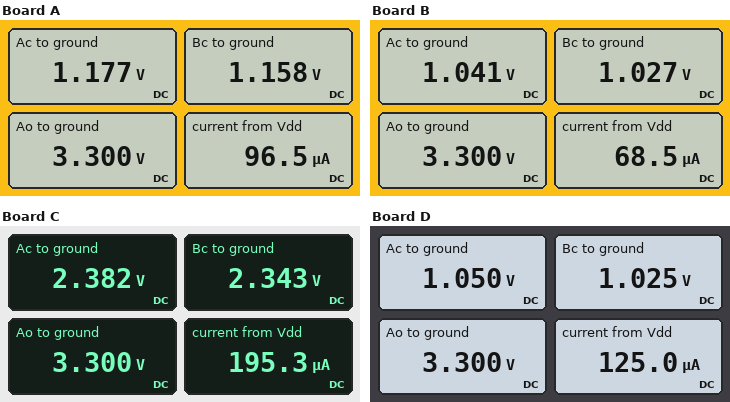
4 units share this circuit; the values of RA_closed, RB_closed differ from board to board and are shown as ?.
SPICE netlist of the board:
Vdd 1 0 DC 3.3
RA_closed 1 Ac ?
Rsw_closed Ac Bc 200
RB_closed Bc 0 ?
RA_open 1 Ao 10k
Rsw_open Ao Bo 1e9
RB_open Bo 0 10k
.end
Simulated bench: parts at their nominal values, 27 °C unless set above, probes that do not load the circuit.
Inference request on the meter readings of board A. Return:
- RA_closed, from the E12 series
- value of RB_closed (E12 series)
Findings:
22 kΩ
12 kΩ
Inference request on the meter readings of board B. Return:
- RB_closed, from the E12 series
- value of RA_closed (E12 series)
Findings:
15 kΩ
33 kΩ
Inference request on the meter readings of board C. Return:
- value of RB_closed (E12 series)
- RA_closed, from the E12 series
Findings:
12 kΩ
4.7 kΩ
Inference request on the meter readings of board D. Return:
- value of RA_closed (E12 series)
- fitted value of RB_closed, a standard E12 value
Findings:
18 kΩ
8.2 kΩ
